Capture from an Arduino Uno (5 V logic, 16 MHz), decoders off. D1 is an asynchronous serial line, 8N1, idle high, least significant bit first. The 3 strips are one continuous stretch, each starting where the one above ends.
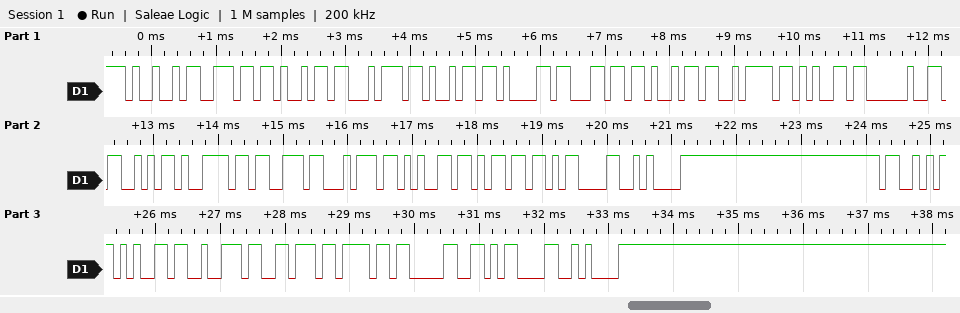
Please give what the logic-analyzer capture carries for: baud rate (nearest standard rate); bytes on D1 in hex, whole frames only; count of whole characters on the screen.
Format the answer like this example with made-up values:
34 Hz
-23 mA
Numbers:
9600 baud
0x49 0x6E 0x69 0x74 0x69 0x61 0x6C 0x69 0x7A 0x65 0x20 0x53 0x79 0x73 0x74 0x65 0x6D 0x0D 0x0A 0x53 0x65 0x72 0x76 0x6F 0x30 0x0D 0x0A
27
